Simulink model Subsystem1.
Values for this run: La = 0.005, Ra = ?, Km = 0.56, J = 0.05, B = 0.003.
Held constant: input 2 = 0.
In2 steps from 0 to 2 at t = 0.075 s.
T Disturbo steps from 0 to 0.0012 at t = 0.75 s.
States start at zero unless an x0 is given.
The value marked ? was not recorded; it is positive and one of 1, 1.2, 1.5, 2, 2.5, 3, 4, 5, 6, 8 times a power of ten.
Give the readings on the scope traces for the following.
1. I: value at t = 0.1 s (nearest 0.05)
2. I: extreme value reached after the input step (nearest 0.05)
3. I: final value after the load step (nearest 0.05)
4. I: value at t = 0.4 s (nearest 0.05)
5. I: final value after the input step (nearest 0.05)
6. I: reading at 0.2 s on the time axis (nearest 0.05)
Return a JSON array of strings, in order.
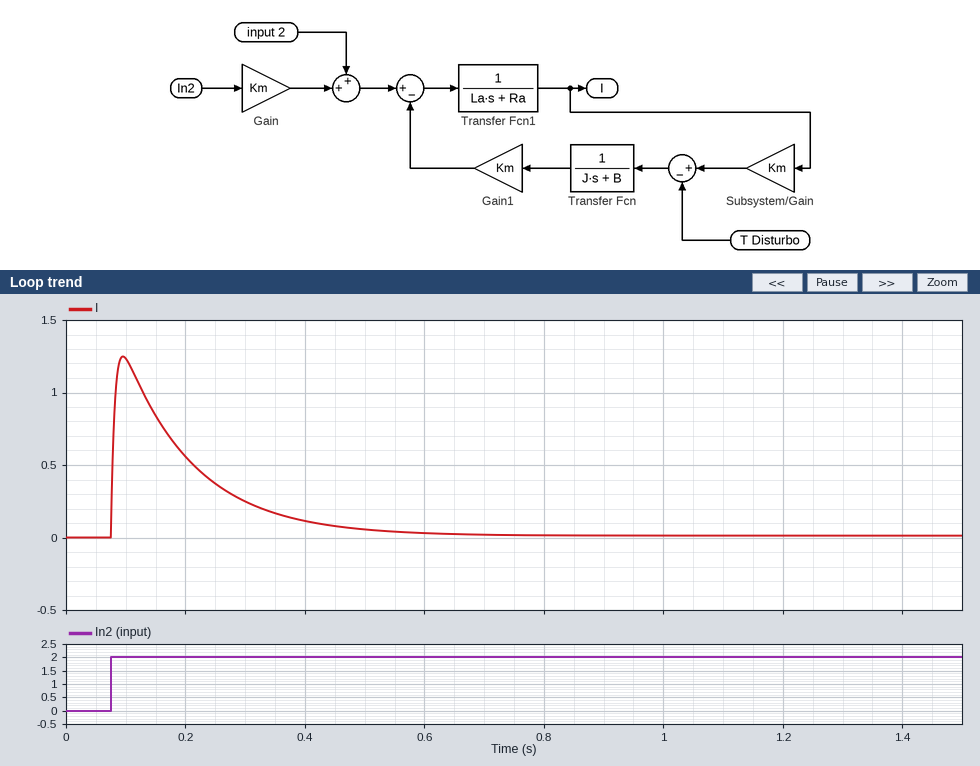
["1.25", "1.25", "0.00", "0.10", "0.00", "0.55"]
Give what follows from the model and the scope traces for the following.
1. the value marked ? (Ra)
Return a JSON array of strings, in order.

["0.8"]
